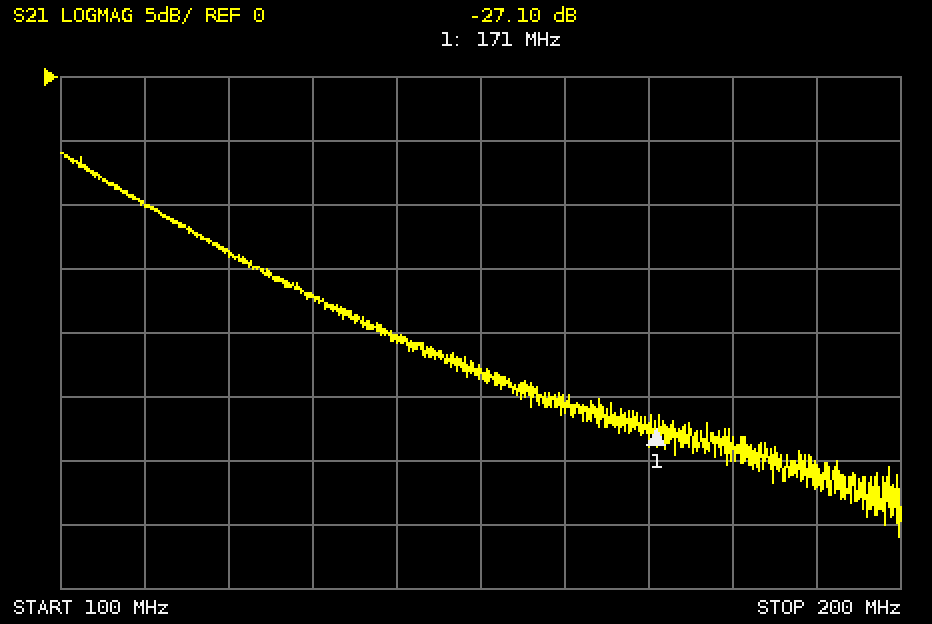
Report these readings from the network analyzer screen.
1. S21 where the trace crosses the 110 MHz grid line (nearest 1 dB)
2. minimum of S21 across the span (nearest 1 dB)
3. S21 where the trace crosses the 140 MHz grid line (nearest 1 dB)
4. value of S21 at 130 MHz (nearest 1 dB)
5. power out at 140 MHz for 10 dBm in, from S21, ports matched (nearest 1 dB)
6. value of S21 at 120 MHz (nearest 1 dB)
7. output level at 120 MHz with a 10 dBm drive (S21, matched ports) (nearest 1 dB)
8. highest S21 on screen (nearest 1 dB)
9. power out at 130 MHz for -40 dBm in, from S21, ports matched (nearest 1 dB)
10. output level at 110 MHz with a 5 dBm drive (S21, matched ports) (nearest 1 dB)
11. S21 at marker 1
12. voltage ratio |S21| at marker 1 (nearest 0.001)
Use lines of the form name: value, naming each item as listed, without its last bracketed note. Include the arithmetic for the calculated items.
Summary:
S21 where the trace crosses the 110 MHz grid line: -10 dB
minimum of S21 across the span: -36 dB
S21 where the trace crosses the 140 MHz grid line: -20 dB
value of S21 at 130 MHz: -17 dB
power out at 140 MHz for 10 dBm in, from S21, ports matched: 10 dBm + (-20 dB) = -10 dBm
value of S21 at 120 MHz: -14 dB
output level at 120 MHz with a 10 dBm drive (S21, matched ports): 10 dBm + (-14 dB) = -4 dBm
highest S21 on screen: -6 dB
power out at 130 MHz for -40 dBm in, from S21, ports matched: -40 dBm + (-17 dB) = -57 dBm
output level at 110 MHz with a 5 dBm drive (S21, matched ports): 5 dBm + (-10 dB) = -5 dBm
S21 at marker 1: -27.10 dB
voltage ratio |S21| at marker 1: 10^(-27.1/20) ≈ 0.044
